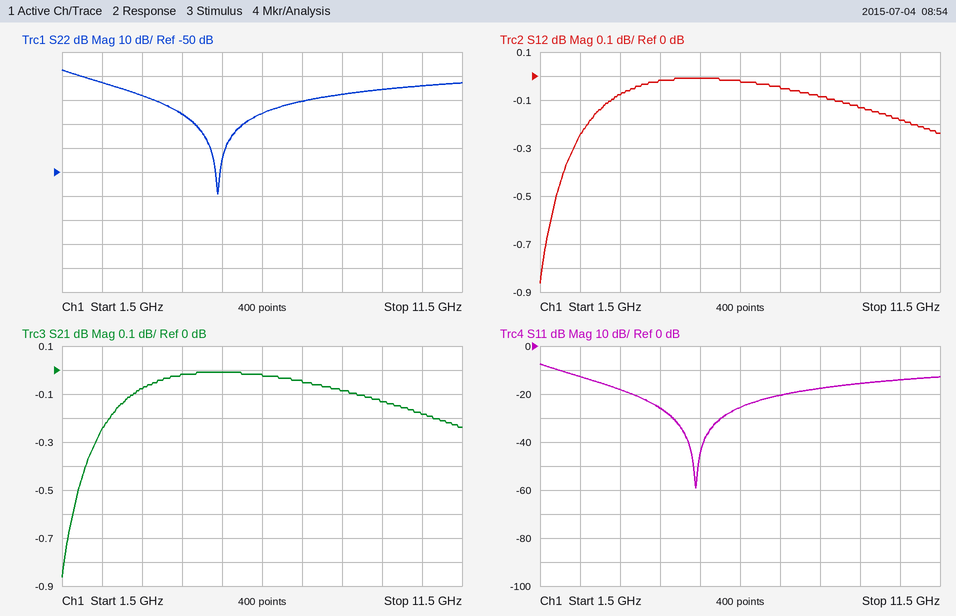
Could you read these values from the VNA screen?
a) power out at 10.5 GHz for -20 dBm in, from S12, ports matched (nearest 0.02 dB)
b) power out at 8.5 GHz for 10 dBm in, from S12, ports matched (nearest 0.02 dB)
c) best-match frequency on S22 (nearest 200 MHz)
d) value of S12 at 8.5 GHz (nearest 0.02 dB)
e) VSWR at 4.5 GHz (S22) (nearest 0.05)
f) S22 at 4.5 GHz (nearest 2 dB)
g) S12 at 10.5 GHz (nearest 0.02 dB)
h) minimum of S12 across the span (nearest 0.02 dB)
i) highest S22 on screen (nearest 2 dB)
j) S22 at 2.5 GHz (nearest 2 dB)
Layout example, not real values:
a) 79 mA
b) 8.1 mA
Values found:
a) -20.18 dBm
b) 9.92 dBm
c) 5.4 GHz
d) -0.08 dB
e) 1.10
f) -26 dB
g) -0.18 dB
h) -0.86 dB
i) -8 dB
j) -12 dB
